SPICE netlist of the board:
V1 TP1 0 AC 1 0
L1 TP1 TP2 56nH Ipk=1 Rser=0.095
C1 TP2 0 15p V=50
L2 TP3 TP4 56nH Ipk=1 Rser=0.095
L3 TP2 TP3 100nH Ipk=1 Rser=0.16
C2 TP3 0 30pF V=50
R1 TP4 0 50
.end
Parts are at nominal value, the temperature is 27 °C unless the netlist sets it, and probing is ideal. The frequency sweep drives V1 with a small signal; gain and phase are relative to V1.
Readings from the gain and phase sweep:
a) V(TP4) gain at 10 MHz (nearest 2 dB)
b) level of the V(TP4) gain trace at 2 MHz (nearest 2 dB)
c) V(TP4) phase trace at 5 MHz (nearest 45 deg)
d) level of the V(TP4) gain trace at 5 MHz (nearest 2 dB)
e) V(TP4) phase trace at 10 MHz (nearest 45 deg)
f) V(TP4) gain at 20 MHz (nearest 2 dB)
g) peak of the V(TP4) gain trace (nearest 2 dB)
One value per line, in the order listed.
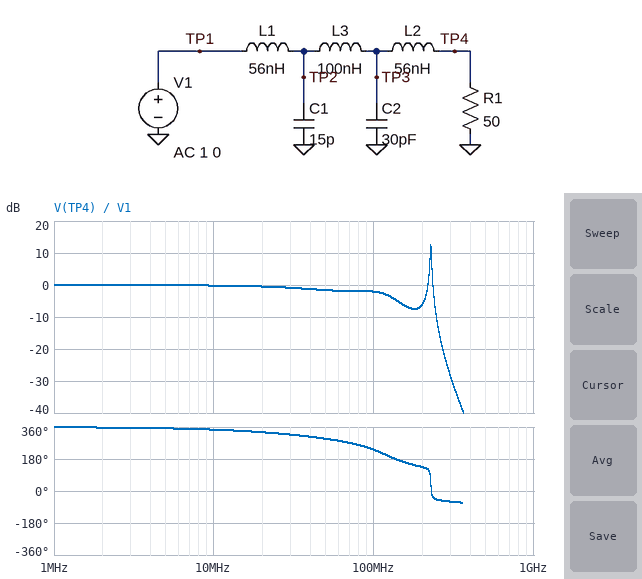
0 dB
0 dB
360 deg
0 dB
360 deg
0 dB
12 dB
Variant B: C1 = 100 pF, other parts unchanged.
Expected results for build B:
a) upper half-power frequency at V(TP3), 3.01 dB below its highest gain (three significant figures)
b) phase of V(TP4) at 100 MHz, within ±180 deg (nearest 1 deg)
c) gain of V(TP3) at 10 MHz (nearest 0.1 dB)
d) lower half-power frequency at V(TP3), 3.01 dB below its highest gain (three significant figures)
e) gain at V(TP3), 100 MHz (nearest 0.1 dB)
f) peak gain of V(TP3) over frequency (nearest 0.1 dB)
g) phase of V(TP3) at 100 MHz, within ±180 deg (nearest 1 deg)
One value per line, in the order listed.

83.6 MHz
112 deg
0 dB
56.6 MHz
0.1 dB
8.1 dB
147 deg
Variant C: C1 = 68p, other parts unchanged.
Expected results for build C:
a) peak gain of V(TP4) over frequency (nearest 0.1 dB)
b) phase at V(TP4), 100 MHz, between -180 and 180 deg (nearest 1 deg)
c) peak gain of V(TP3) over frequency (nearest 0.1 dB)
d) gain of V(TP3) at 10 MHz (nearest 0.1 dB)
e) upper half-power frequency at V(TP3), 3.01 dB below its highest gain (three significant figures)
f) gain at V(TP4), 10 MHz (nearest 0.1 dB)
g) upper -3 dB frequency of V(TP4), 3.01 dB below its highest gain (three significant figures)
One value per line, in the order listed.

5.4 dB
150 deg
6.7 dB
0 dB
109 MHz
-0.1 dB
106 MHz
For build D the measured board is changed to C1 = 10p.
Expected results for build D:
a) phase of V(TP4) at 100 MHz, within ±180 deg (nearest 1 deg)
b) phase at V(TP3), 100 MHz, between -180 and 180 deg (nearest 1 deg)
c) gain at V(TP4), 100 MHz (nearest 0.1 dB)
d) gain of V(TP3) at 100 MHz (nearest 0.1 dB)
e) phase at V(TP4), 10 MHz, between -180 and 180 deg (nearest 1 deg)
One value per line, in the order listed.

-126 deg
-91 deg
-2.8 dB
-1.0 dB
-15 deg
